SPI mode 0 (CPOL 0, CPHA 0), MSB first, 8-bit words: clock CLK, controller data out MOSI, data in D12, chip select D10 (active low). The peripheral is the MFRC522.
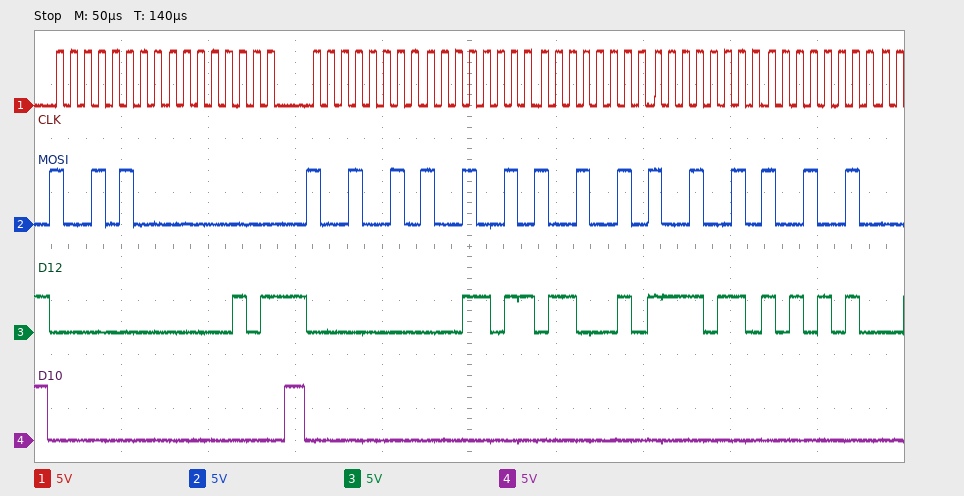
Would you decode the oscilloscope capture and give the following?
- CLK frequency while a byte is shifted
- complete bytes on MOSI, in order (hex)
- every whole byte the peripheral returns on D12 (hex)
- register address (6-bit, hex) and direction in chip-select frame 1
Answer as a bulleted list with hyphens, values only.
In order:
- 125 kHz
- 94 00 92 92 92 92 92
- 00 05 00 1B 62 F6 AA
- 0x0A read
